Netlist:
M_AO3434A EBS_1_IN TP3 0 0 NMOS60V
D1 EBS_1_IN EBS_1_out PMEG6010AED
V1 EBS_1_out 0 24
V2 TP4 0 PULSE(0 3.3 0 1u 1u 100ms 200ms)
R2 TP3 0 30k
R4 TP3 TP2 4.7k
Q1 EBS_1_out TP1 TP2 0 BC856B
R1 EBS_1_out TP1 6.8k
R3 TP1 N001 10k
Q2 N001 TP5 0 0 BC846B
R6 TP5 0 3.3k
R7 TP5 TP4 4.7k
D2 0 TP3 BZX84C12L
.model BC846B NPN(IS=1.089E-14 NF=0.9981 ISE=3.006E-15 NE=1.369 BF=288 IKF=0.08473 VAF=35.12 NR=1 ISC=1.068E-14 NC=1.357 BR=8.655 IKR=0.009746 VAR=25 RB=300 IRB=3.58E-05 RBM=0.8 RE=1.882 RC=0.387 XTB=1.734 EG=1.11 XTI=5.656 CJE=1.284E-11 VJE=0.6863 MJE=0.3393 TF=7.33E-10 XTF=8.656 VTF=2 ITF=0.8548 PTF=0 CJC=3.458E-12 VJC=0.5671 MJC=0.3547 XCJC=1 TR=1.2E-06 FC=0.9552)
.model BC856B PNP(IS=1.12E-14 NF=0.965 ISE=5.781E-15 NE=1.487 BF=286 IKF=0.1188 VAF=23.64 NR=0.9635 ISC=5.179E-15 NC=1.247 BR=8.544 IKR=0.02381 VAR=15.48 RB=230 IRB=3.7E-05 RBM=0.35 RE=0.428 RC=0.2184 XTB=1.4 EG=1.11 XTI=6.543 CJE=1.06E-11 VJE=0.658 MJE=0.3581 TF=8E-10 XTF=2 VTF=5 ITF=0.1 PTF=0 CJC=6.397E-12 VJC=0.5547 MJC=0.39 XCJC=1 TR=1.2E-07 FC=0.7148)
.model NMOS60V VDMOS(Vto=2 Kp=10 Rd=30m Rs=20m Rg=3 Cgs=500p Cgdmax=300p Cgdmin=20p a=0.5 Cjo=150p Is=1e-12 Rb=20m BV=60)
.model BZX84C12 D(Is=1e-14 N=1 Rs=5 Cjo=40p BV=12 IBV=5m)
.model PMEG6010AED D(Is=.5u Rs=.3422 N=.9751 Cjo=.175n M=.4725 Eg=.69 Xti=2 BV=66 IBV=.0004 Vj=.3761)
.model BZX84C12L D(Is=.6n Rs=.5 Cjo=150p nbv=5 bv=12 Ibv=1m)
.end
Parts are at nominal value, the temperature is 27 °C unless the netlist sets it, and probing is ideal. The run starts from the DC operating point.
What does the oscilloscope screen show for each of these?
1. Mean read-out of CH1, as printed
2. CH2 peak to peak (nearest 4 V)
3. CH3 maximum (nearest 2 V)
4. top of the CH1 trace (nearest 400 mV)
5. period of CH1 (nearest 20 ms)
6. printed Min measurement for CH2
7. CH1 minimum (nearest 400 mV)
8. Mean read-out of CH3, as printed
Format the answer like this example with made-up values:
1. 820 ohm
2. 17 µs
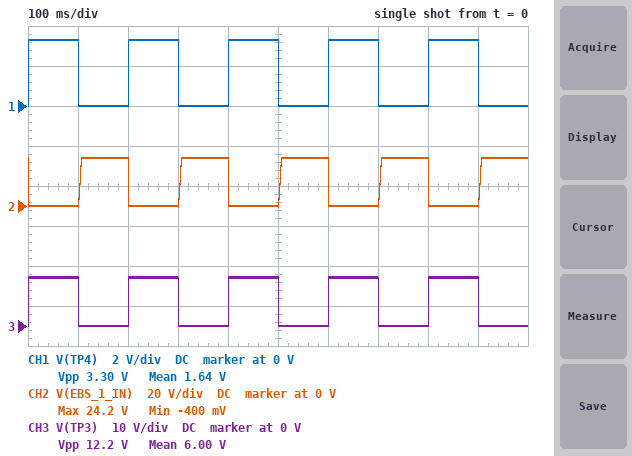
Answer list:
1. 1.64 V
2. 24 V
3. 12 V
4. 3.2 V
5. 200 ms
6. -400 mV
7. 0 V
8. 6.00 V
